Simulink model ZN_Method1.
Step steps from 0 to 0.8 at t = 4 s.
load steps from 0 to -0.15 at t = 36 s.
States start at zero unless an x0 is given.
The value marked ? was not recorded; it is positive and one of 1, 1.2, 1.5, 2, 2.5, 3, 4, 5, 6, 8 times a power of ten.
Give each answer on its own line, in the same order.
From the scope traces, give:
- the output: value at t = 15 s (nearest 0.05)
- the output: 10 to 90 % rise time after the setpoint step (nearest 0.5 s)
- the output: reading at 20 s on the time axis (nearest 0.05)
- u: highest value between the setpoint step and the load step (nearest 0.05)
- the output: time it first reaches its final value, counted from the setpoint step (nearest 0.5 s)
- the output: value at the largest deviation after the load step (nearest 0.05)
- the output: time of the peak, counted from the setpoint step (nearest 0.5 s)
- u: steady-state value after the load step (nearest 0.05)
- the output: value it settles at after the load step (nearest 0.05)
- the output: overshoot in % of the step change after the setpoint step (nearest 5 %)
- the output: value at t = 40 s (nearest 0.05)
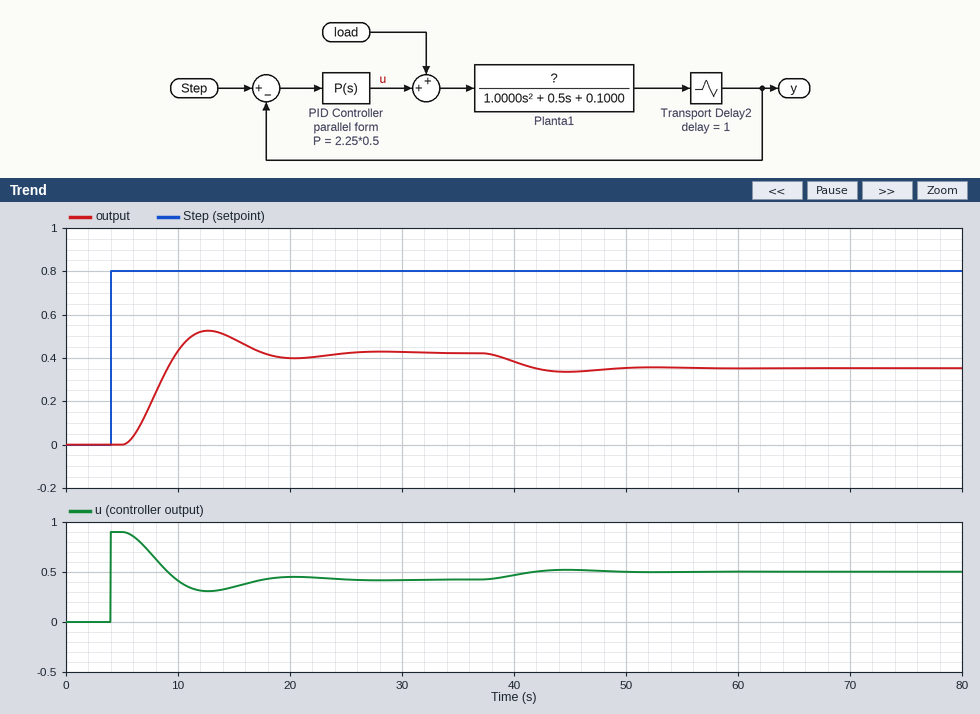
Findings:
0.50
3.5 s
0.40
0.90
6.0 s
0.35
8.5 s
0.50
0.35
25 %
0.40
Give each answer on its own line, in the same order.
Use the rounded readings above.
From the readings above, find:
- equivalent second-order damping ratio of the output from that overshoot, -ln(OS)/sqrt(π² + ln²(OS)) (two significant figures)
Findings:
0.40
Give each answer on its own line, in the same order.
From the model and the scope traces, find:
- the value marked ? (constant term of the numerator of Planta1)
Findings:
0.1
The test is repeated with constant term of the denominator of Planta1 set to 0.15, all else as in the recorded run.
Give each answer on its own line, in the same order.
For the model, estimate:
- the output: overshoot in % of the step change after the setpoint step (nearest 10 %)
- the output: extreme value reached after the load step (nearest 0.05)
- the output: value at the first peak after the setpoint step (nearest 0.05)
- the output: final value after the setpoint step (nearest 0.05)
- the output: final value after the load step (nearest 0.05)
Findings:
30 %
0.25
0.45
0.35
0.30
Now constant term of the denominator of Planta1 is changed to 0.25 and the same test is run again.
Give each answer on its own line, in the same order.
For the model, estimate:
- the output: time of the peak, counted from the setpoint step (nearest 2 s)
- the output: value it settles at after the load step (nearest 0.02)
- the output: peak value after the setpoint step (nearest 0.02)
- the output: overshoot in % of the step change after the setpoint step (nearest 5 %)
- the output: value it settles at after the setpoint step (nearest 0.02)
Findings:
6 s
0.20
0.34
35 %
0.24
